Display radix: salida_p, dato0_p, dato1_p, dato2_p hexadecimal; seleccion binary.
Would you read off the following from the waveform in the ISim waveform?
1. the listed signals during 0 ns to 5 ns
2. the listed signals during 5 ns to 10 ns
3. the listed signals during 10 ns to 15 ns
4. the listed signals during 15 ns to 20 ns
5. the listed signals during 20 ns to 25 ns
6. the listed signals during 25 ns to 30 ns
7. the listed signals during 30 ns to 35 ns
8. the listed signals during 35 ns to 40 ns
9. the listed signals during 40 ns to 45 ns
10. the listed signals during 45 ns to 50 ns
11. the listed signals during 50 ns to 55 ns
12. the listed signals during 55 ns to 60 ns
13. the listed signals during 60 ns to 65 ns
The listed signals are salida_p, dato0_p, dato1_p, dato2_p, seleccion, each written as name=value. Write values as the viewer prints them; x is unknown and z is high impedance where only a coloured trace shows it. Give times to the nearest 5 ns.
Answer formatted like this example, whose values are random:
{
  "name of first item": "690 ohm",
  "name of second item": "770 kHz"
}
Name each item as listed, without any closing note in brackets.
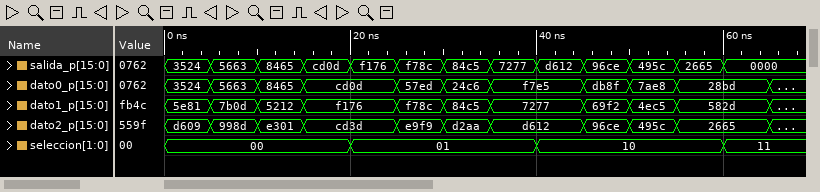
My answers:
{
  "the listed signals during 0 ns to 5 ns": "salida_p=3524, dato0_p=3524, dato1_p=5e81, dato2_p=d609, seleccion=00",
  "the listed signals during 5 ns to 10 ns": "salida_p=5663, dato0_p=5663, dato1_p=7b0d, dato2_p=998d, seleccion=00",
  "the listed signals during 10 ns to 15 ns": "salida_p=8465, dato0_p=8465, dato1_p=5212, dato2_p=e301, seleccion=00",
  "the listed signals during 15 ns to 20 ns": "salida_p=cd0d, dato0_p=cd0d, dato1_p=f176, dato2_p=cd3d, seleccion=00",
  "the listed signals during 20 ns to 25 ns": "salida_p=f176, dato0_p=cd0d, dato1_p=f176, dato2_p=cd3d, seleccion=01",
  "the listed signals during 25 ns to 30 ns": "salida_p=f78c, dato0_p=57ed, dato1_p=f78c, dato2_p=e9f9, seleccion=01",
  "the listed signals during 30 ns to 35 ns": "salida_p=84c5, dato0_p=24c6, dato1_p=84c5, dato2_p=d2aa, seleccion=01",
  "the listed signals during 35 ns to 40 ns": "salida_p=7277, dato0_p=f7e5, dato1_p=7277, dato2_p=d612, seleccion=01",
  "the listed signals during 40 ns to 45 ns": "salida_p=d612, dato0_p=f7e5, dato1_p=7277, dato2_p=d612, seleccion=10",
  "the listed signals during 45 ns to 50 ns": "salida_p=96ce, dato0_p=db8f, dato1_p=69f2, dato2_p=96ce, seleccion=10",
  "the listed signals during 50 ns to 55 ns": "salida_p=495c, dato0_p=7ae8, dato1_p=4ec5, dato2_p=495c, seleccion=10",
  "the listed signals during 55 ns to 60 ns": "salida_p=2665, dato0_p=28bd, dato1_p=582d, dato2_p=2665, seleccion=10",
  "the listed signals during 60 ns to 65 ns": "salida_p=0000, dato0_p=28bd, dato1_p=582d, dato2_p=2665, seleccion=11"
}
